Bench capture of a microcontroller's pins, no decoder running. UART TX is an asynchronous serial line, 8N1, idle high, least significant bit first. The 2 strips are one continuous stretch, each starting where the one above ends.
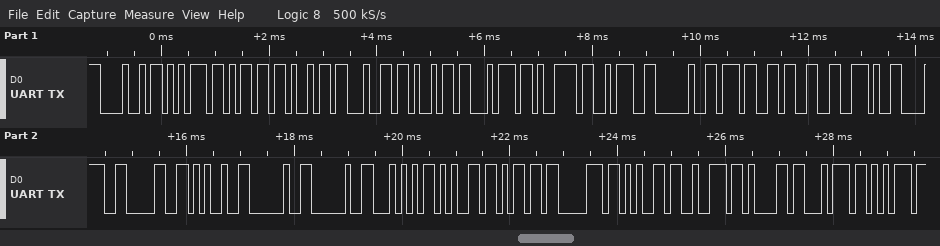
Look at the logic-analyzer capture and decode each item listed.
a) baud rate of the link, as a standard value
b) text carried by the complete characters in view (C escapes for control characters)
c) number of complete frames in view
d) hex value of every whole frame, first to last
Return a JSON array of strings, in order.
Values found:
["9600 baud", "\"Humidity: 73.80%  Temperatu\"", "27", "48 75 6D 69 64 69 74 79 3A 20 37 33 2E 38 30 25 20 20 54 65 6D 70 65 72 61 74 75"]
